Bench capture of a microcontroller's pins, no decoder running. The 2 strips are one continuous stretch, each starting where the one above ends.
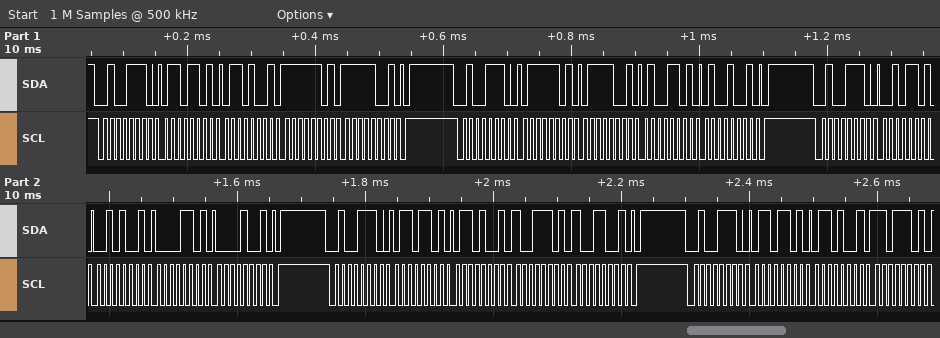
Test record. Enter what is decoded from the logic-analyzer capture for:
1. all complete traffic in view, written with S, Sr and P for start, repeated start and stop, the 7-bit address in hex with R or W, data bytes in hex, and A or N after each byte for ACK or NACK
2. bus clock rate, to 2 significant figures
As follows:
S 27W A 6D A 69 A FD A F9 A P S 27W A 7D A 79 A 4D A 49 A P S 27W A 2D A 29 A 0D A 09 A P S 27W A 6D A 69 A 9D A 99 A P S 27W A 6D A 69 A DD A
100 kHz
